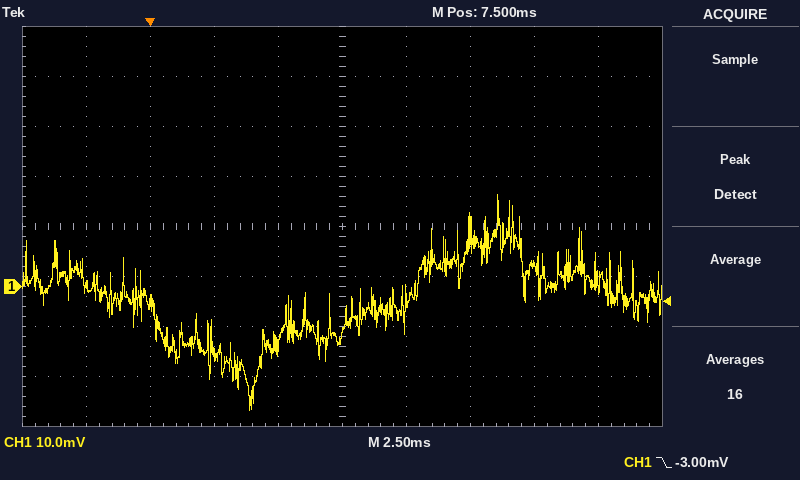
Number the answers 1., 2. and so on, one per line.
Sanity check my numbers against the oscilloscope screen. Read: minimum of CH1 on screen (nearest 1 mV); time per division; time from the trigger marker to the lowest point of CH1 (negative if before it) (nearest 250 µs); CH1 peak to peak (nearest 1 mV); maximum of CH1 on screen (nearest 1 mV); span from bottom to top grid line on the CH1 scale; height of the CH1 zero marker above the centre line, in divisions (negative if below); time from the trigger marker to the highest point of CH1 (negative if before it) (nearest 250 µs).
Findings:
1. -25 mV
2. 2.5 ms
3. +4.00 ms
4. 43 mV
5. 18 mV
6. 80 mV
7. -1.2 div
8. +13.50 ms
